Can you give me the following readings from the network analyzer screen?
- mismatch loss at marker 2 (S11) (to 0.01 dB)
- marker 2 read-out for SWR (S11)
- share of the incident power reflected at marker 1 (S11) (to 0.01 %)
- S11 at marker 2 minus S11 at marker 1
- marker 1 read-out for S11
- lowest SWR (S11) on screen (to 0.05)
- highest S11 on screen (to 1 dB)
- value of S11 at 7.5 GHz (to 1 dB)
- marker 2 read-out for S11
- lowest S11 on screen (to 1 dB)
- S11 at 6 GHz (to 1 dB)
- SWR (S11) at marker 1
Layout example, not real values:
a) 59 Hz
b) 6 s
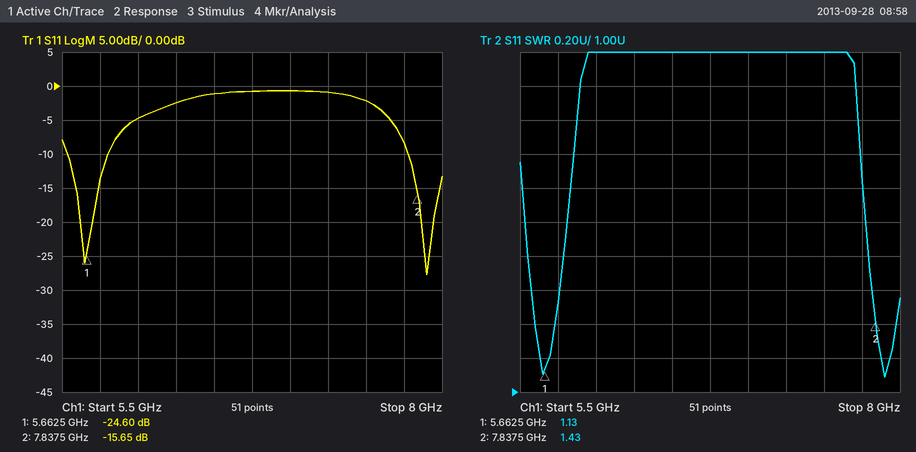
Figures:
a) 0.12 dB
b) 1.43
c) 0.35 %
d) 8.95 dB
e) -24.60 dB
f) 1.10
g) -1 dB
h) -2 dB
i) -15.65 dB
j) -28 dB
k) -5 dB
l) 1.13
